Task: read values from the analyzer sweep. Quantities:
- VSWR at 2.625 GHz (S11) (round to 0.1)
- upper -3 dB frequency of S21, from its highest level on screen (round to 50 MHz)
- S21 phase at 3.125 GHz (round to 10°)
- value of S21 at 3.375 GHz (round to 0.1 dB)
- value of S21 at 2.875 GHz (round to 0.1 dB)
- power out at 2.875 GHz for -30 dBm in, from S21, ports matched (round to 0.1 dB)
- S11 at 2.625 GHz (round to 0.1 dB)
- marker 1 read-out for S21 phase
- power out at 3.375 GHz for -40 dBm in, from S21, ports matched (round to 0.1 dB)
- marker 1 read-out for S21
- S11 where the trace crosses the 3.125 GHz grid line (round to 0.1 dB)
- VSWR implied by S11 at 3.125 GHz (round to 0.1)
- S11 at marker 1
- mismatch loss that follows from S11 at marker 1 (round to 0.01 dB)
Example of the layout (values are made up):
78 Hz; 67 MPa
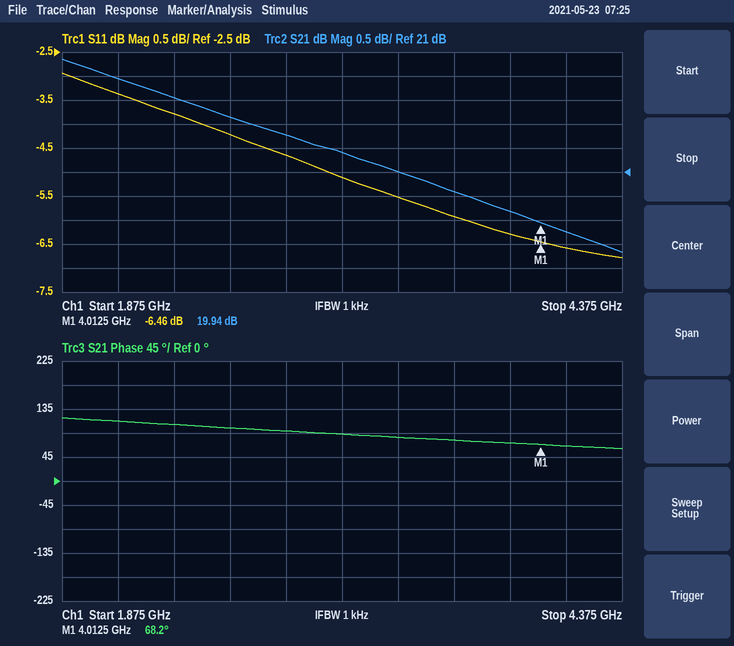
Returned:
4.2; 3.75 GHz; 90°; 21.0 dB; 21.8 dB; -8.2 dBm; -4.2 dB; 68.2°; -19.0 dBm; 19.94 dB; -5.1 dB; 3.5; -6.46 dB; 1.11 dB
